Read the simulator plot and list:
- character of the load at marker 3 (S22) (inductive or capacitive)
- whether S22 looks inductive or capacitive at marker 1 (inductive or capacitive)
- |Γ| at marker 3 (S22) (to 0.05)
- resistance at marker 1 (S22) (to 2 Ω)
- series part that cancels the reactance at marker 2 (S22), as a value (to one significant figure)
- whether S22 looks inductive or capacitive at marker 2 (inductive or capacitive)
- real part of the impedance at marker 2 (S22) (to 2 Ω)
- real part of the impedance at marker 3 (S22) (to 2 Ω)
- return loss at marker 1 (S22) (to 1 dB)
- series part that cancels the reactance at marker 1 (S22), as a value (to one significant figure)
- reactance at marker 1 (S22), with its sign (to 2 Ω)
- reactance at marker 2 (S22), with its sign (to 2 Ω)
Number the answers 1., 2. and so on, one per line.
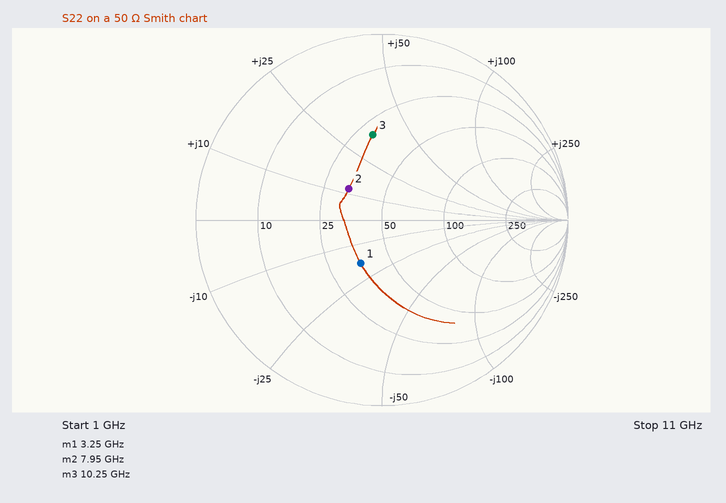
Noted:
1. inductive
2. capacitive
3. 0.45
4. 36 Ω
5. 2 pF
6. inductive
7. 34 Ω
8. 30 Ω
9. 12 dB
10. 900 pH
11. -18 Ω
12. +12 Ω
